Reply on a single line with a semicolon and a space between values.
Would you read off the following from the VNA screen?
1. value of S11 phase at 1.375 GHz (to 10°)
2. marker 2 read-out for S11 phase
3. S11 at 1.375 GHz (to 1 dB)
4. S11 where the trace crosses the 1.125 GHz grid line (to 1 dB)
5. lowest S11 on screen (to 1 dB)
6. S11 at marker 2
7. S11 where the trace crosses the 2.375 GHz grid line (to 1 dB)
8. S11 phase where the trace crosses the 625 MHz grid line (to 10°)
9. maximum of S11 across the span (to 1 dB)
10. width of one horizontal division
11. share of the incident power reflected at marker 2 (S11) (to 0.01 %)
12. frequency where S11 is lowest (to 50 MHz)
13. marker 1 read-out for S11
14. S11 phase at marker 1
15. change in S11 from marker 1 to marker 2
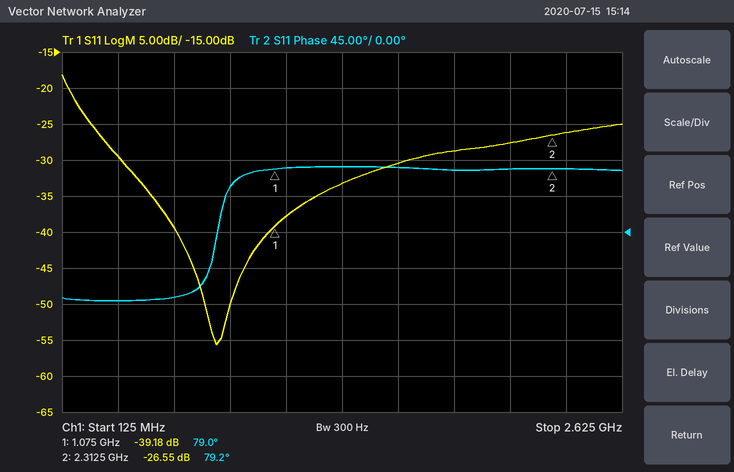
80°; 79.2°; -33 dB; -38 dB; -56 dB; -26.55 dB; -26 dB; -80°; -18 dB; 250 MHz; 0.22 %; 800 MHz; -39.18 dB; 79.0°; 12.63 dB
